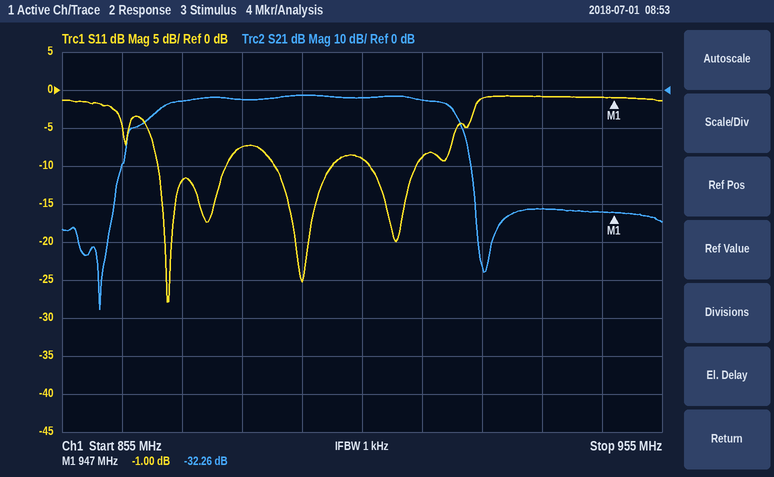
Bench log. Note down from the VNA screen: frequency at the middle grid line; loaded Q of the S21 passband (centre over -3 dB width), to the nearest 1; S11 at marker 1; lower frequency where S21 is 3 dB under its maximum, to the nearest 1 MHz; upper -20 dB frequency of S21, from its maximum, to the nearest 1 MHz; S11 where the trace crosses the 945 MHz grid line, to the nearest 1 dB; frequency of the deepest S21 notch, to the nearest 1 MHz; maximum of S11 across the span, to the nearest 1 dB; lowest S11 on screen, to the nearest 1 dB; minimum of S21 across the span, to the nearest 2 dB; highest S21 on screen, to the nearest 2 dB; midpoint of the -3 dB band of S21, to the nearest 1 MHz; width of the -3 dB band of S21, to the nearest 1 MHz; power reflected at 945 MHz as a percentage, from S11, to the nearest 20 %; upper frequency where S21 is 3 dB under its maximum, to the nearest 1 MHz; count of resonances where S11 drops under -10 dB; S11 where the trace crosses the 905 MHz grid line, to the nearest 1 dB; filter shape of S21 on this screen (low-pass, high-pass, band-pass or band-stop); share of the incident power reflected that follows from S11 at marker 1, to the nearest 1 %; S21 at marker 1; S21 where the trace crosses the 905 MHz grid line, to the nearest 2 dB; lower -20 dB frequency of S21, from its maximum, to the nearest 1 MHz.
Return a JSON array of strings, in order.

["905 MHz", "19", "-1.00 dB", "872 MHz", "923 MHz", "-1 dB", "861 MHz", "-1 dB", "-28 dB", "-58 dB", "-2 dB", "896 MHz", "48 MHz", "80 %", "920 MHz", "4", "-9 dB", "band-pass", "79 %", "-32.26 dB", "-2 dB", "865 MHz"]
